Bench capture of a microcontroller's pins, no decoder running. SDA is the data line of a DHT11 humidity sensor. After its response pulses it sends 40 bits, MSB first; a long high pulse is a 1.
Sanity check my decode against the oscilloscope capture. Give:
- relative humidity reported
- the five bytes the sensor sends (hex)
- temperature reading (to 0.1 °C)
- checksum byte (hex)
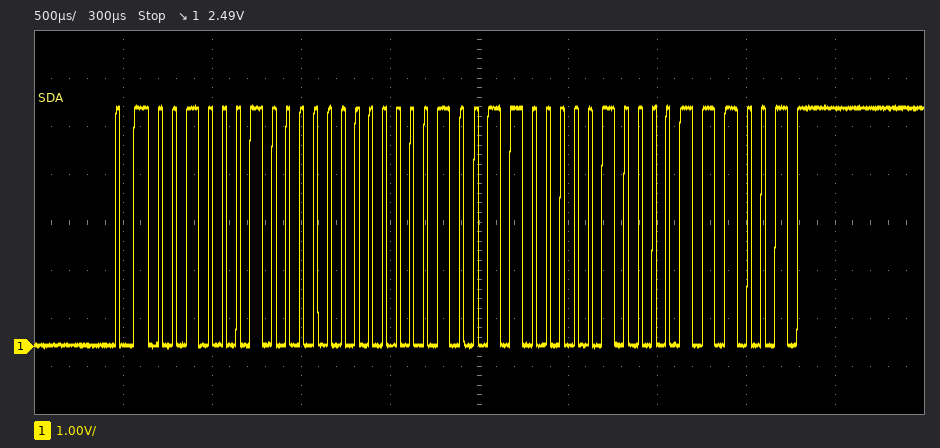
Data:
34 %
22 00 13 04 39
19.4 °C
0x39
